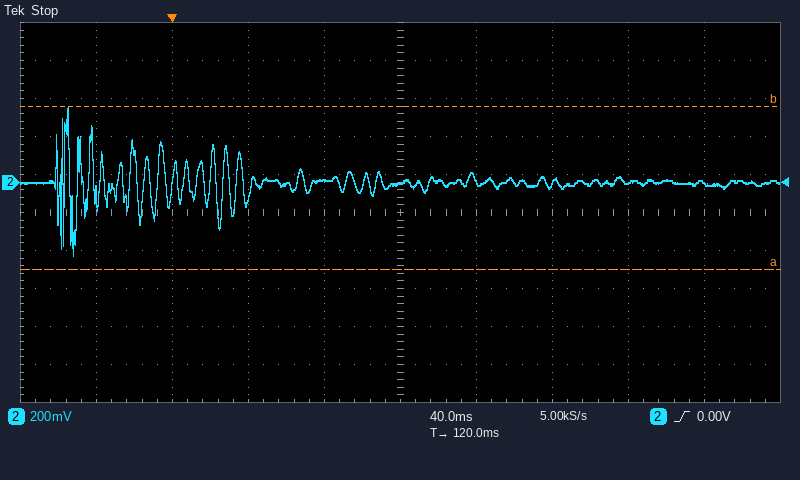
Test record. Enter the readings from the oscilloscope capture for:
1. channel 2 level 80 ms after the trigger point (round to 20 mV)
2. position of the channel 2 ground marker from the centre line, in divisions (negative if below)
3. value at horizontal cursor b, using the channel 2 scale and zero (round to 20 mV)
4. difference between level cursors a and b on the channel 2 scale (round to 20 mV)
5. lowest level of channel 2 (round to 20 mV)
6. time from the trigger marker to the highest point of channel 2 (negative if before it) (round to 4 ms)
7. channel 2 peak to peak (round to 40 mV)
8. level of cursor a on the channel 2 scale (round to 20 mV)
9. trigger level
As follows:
20 mV
+0.8 div
400 mV
860 mV
-380 mV
-56 ms
760 mV
-460 mV
0.00 V
